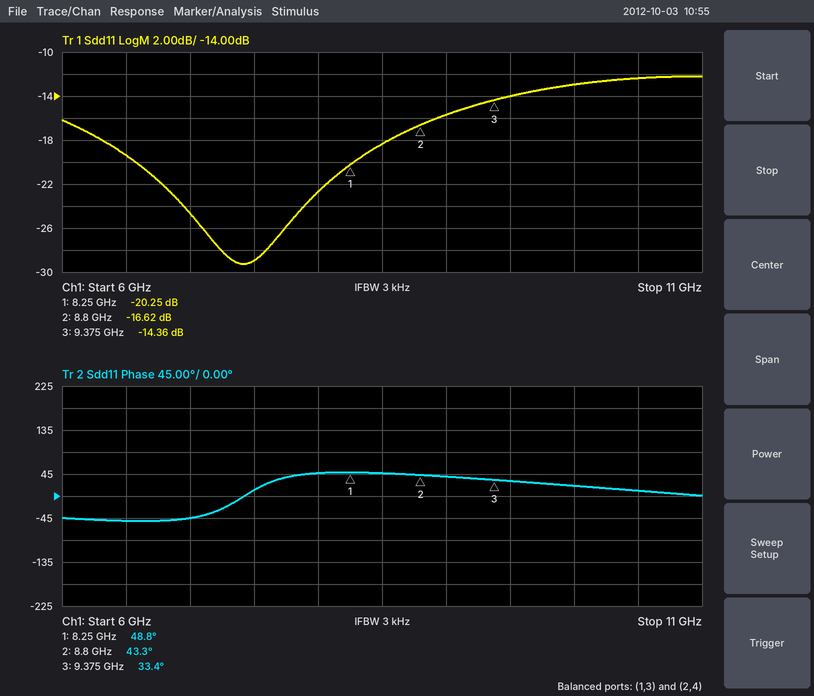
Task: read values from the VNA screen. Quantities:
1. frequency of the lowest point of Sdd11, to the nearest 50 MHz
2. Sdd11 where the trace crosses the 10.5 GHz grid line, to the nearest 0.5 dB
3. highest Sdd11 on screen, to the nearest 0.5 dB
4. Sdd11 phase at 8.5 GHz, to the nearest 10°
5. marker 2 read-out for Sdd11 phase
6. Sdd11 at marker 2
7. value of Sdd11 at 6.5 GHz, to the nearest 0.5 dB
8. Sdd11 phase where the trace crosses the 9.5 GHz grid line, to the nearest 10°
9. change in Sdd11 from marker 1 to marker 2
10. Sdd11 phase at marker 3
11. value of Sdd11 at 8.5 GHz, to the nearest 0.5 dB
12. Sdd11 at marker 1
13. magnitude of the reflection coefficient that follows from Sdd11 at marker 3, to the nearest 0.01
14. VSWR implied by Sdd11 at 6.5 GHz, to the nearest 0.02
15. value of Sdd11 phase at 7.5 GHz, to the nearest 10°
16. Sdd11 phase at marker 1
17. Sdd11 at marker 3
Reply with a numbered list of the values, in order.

1. 7.40 GHz
2. -12.5 dB
3. -12.0 dB
4. 50°
5. 43.3°
6. -16.62 dB
7. -19.5 dB
8. 30°
9. 3.63 dB
10. 33.4°
11. -18.5 dB
12. -20.25 dB
13. 0.19
14. 1.24
15. 10°
16. 48.8°
17. -14.36 dB
